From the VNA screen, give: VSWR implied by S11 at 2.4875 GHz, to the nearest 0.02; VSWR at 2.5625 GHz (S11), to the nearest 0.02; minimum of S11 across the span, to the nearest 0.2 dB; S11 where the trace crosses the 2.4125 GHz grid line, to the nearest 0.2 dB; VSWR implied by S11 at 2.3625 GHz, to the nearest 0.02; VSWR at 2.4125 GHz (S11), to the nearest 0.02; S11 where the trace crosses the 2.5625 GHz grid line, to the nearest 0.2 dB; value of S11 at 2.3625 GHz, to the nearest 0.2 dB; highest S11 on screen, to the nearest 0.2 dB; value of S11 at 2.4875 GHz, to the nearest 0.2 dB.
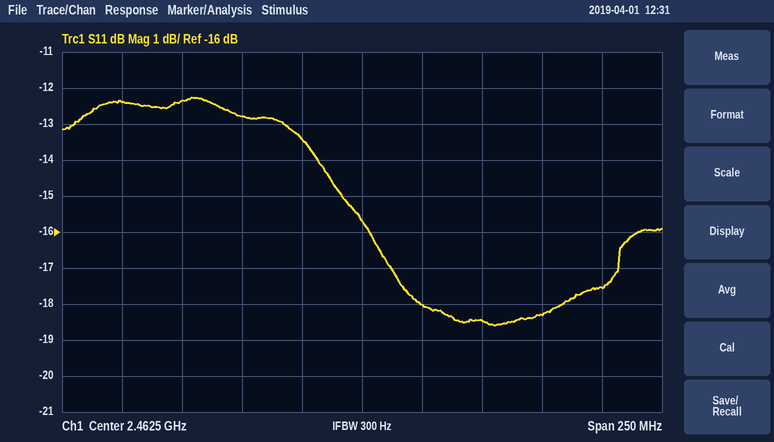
1.28
1.30
-18.6 dB
-12.8 dB
1.64
1.60
-17.6 dB
-12.4 dB
-12.2 dB
-18.0 dB
